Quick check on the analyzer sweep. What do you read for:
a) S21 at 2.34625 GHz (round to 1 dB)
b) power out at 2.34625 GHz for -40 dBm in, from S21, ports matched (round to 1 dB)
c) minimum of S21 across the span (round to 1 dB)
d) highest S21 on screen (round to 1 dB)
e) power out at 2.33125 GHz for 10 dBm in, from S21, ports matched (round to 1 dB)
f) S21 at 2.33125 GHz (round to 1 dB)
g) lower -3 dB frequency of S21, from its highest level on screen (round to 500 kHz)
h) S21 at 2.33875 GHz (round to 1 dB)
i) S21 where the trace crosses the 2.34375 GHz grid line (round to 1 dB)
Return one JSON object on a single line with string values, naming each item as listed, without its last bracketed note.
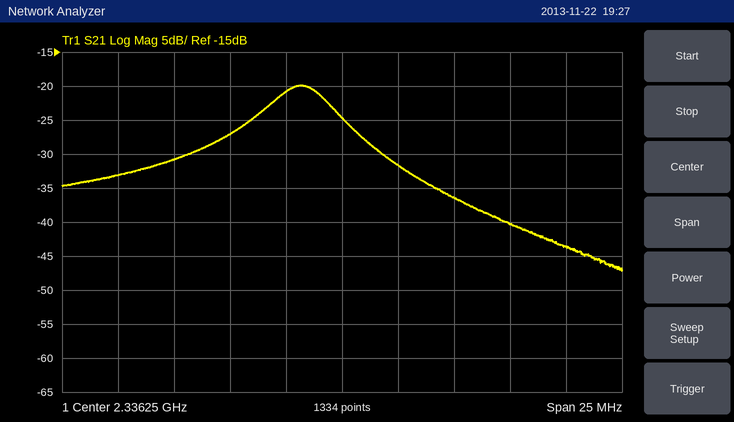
{"S21 at 2.34625 GHz": "-44 dB", "power out at 2.34625 GHz for -40 dBm in, from S21, ports matched": "-84 dBm", "minimum of S21 across the span": "-47 dB", "highest S21 on screen": "-20 dB", "power out at 2.33125 GHz for 10 dBm in, from S21, ports matched": "-17 dBm", "S21 at 2.33125 GHz": "-27 dB", "lower -3 dB frequency of S21, from its highest level on screen": "2.3330 GHz", "S21 at 2.33875 GHz": "-32 dB", "S21 where the trace crosses the 2.34375 GHz grid line": "-40 dB"}
